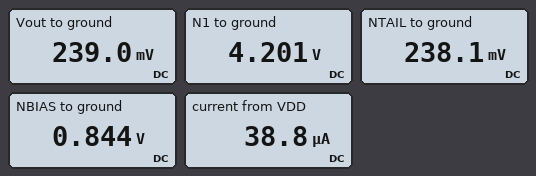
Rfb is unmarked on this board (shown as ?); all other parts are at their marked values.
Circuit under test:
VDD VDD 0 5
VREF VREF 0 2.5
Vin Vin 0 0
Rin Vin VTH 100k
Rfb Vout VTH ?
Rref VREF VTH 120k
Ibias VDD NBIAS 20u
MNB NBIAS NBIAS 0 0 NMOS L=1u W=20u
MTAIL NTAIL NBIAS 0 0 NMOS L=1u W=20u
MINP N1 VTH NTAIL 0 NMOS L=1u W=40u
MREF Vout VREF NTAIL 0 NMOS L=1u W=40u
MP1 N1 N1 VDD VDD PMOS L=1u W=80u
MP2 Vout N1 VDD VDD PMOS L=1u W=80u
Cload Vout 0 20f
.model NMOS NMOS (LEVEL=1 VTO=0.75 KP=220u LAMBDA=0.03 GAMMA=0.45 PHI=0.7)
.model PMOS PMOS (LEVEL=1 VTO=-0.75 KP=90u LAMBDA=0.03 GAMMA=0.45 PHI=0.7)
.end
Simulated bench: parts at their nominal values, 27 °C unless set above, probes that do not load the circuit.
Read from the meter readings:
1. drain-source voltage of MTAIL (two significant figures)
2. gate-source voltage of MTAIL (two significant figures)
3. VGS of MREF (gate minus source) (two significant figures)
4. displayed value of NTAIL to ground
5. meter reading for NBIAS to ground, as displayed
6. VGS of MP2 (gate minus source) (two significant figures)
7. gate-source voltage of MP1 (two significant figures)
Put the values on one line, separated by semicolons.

240 mV; 840 mV; 2.3 V; 238.1 mV; 0.844 V; -800 mV; -800 mV
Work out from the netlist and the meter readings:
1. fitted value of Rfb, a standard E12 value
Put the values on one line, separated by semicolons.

1 MΩ
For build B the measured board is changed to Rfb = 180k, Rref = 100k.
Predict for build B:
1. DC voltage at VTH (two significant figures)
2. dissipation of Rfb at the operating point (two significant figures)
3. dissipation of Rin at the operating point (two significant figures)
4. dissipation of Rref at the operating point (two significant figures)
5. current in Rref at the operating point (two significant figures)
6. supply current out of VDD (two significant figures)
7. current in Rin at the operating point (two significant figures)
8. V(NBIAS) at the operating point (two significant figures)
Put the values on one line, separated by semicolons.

1.0 V; 3.9 µW; 10 µW; 22 µW; 15 µA; 35 µA; 10 µA; 840 mV
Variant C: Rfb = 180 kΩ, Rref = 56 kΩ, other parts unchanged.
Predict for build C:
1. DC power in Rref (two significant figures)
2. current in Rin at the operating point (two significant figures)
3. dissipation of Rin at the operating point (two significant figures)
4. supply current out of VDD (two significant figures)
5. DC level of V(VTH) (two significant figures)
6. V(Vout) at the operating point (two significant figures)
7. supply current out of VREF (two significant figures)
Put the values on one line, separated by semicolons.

21 µW; 14 µA; 20 µW; 35 µA; 1.4 V; 520 mV; 19 µA
